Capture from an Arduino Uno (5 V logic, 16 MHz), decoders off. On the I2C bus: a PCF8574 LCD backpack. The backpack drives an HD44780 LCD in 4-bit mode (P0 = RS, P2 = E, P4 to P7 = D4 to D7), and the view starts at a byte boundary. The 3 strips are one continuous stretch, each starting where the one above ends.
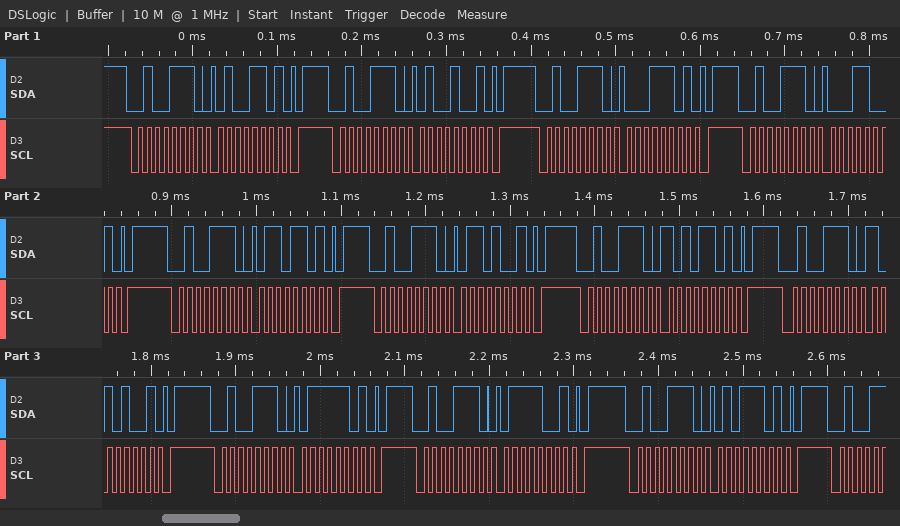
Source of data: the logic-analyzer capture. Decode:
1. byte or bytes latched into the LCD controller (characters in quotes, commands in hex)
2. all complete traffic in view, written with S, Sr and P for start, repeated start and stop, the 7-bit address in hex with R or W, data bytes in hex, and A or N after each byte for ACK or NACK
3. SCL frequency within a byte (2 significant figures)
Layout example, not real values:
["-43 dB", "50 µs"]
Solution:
["'A' 'j'", "S 27W A 4D A P S 27W A 49 A P S 27W A 1D A P S 27W A 19 A P S 27W A 6D A P S 27W A 69 A P S 27W A AD A P S 27W A A9 A P S 27W A 7D A P S 27W A 79 A P S 27W A 5D A P", "100 kHz"]
